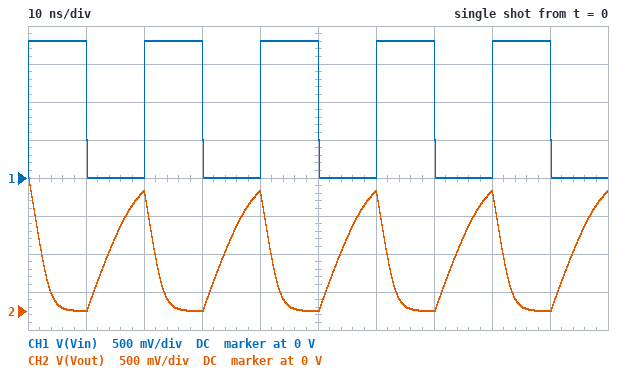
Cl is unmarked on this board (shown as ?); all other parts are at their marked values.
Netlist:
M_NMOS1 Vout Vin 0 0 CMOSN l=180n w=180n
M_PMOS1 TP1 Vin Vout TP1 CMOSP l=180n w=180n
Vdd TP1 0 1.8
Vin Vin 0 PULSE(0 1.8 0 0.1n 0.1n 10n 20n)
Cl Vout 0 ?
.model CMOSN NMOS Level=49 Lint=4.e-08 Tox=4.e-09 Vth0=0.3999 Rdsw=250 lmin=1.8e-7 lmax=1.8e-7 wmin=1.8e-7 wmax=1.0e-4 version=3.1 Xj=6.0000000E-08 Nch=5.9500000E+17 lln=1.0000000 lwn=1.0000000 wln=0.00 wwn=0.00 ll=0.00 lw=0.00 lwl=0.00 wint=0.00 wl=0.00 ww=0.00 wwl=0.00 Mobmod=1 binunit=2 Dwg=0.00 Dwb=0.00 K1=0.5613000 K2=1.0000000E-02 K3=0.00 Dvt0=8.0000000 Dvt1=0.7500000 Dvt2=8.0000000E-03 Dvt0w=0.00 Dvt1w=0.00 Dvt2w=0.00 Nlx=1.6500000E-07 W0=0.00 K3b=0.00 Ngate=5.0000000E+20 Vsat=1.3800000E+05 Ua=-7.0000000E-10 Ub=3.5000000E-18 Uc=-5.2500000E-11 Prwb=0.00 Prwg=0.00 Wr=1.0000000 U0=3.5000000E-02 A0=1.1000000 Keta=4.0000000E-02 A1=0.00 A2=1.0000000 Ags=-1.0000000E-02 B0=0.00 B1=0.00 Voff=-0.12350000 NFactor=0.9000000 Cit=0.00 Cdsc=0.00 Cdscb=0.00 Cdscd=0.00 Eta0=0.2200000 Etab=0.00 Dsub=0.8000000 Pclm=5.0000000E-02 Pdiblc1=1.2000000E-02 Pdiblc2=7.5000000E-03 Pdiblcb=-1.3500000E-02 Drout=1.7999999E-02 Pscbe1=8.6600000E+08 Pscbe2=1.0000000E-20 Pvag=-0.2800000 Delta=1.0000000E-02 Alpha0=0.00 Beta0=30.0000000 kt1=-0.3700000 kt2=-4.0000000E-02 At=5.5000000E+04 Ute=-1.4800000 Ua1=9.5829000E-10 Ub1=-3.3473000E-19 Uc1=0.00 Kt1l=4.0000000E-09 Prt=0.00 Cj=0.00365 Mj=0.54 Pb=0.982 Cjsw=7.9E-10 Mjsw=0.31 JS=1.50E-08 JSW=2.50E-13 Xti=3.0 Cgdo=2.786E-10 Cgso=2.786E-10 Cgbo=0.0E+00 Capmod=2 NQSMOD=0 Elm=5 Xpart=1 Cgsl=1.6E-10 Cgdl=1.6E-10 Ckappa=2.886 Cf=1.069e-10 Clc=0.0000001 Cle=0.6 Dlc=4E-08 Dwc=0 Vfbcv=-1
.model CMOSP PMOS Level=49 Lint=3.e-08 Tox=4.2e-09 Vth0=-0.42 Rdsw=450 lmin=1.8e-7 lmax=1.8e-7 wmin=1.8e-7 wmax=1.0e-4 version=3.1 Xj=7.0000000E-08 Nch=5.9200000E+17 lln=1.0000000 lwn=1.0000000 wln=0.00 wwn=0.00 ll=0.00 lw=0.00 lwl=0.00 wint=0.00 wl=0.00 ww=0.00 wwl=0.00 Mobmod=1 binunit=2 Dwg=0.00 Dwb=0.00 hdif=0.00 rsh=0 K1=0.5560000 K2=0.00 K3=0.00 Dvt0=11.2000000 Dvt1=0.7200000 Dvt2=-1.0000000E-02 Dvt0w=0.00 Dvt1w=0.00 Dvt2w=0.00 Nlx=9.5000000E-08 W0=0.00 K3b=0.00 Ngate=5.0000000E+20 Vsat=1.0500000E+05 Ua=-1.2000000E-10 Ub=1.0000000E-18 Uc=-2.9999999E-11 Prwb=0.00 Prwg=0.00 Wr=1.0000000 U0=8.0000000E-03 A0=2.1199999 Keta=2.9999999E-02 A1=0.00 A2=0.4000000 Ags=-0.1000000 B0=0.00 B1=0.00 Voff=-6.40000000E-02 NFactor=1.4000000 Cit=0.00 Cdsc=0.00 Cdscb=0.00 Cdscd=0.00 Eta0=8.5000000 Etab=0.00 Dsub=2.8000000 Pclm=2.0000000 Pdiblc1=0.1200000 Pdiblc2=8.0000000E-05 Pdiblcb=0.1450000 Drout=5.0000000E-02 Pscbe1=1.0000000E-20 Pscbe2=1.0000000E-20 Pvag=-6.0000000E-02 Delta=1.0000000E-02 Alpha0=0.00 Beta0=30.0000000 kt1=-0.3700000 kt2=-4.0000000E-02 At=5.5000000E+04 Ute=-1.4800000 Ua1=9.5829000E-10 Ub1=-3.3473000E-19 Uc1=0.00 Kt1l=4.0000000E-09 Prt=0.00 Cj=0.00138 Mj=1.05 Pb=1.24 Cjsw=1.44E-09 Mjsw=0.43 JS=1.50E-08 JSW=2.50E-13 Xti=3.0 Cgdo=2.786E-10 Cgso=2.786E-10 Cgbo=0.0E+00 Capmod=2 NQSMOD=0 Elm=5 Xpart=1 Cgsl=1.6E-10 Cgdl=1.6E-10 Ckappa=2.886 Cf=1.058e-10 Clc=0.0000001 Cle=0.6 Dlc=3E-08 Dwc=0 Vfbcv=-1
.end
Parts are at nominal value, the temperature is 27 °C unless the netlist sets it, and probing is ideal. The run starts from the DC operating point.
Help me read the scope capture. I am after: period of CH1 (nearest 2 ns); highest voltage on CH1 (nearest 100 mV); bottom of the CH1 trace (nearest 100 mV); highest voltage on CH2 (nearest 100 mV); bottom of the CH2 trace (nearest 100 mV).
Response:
20 ns
1.8 V
0 V
1.8 V
0 V
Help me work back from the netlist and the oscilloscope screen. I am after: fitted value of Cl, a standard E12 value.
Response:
270 fF
